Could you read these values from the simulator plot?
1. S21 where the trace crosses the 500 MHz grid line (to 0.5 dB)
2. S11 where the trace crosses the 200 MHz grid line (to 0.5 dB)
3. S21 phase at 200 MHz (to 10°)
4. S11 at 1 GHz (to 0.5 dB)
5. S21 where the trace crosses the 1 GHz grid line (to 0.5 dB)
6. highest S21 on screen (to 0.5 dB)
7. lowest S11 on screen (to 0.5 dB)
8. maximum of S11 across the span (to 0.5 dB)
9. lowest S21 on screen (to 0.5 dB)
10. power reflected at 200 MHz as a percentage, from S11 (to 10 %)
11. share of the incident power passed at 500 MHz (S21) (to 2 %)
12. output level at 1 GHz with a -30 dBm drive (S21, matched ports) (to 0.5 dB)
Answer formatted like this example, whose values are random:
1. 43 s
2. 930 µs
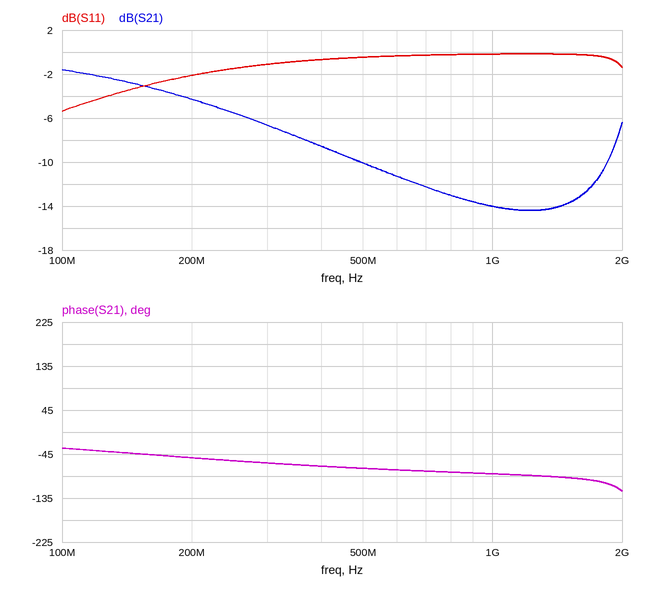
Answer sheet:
1. -10.0 dB
2. -2.0 dB
3. -50°
4. 0.0 dB
5. -14.0 dB
6. -1.5 dB
7. -5.5 dB
8. 0.0 dB
9. -14.5 dB
10. 60 %
11. 10 %
12. -44.0 dBm
